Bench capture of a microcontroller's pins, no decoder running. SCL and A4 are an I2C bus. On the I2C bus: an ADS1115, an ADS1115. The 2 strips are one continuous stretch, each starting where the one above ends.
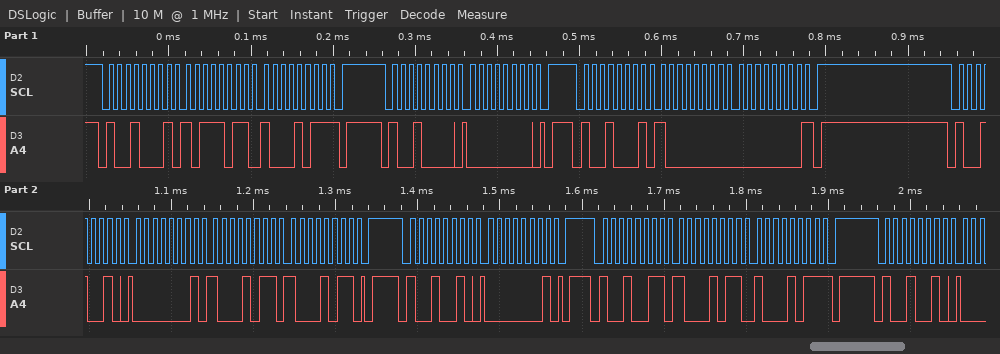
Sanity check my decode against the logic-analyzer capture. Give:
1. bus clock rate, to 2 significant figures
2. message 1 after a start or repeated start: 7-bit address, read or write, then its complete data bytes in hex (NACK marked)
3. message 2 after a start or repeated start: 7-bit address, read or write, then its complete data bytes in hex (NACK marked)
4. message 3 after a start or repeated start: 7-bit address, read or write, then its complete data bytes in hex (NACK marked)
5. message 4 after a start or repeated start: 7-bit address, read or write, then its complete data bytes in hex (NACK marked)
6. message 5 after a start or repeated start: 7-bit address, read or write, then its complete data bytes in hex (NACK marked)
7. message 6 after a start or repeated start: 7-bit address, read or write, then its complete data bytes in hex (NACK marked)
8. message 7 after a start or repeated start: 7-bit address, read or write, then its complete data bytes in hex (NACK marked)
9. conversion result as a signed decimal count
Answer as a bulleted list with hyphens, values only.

- 100 kHz
- 0x48 read: BB 8B NACK
- 0x48 write: 00
- 0x48 read: 80 00 NACK
- 0x49 write: 01 8B 8B
- 0x49 write: 01
- 0x49 read: 8B 8B NACK
- 0x49 write
- -32768
